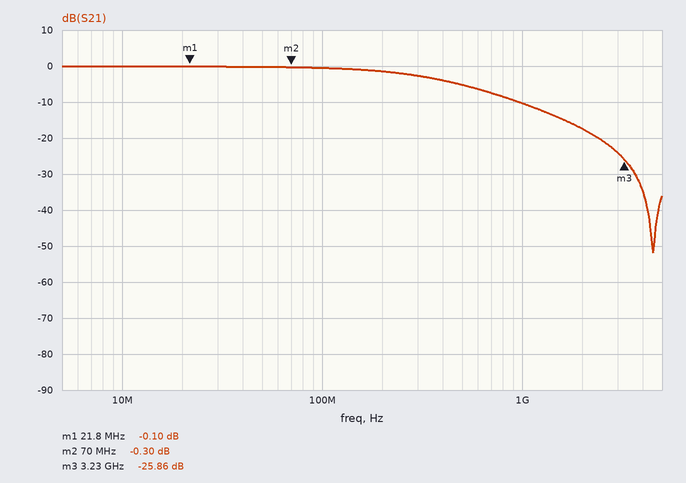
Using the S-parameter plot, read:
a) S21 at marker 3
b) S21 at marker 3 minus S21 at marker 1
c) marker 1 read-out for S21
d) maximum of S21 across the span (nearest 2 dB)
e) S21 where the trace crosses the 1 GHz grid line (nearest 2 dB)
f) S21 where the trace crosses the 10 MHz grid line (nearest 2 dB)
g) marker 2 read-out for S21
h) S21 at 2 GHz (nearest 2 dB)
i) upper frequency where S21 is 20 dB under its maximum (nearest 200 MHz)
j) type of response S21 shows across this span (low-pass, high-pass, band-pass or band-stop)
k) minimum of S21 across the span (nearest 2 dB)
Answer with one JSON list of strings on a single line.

["-25.86 dB", "-25.76 dB", "-0.10 dB", "0 dB", "-10 dB", "0 dB", "-0.30 dB", "-18 dB", "2.4 GHz", "low-pass", "-52 dB"]
